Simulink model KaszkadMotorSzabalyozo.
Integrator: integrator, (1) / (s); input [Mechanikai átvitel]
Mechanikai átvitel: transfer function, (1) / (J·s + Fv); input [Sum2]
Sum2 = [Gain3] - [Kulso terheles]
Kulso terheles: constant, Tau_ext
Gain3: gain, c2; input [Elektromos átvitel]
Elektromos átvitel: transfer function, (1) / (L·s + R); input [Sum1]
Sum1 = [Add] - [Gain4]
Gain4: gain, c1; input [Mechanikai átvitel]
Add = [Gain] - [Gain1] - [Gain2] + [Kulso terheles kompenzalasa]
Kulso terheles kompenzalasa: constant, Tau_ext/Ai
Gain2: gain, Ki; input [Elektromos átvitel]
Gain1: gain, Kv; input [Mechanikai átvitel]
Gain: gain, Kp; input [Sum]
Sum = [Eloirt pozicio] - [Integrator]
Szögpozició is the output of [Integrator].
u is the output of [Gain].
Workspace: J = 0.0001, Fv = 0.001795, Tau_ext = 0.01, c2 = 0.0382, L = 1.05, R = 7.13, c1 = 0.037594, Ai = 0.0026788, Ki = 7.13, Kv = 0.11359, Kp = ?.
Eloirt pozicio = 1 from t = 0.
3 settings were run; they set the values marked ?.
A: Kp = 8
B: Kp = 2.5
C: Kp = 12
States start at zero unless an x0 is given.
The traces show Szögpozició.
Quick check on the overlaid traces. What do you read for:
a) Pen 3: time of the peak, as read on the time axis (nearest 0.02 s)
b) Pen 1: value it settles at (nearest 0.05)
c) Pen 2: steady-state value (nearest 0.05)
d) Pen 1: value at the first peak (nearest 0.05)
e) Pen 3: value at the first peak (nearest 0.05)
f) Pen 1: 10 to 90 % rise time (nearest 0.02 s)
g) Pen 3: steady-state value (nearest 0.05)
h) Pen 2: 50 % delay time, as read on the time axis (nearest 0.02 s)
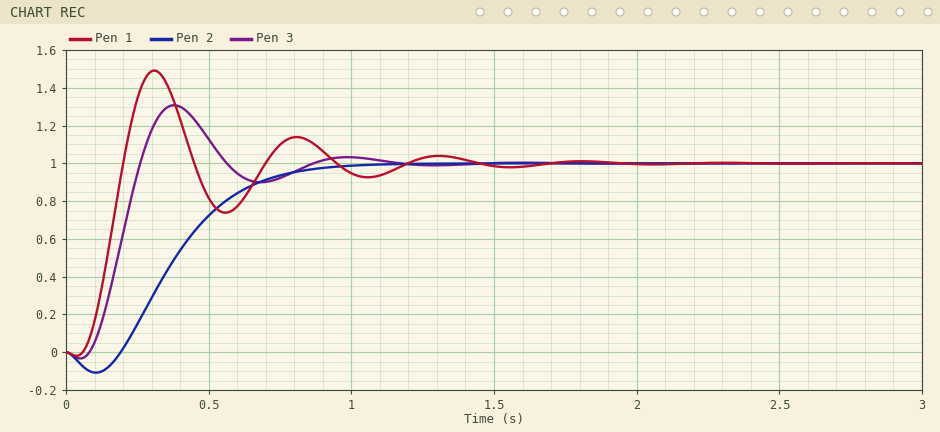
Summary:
0.38 s
1.00
1.00
1.50
1.30
0.10 s
1.00
0.38 s
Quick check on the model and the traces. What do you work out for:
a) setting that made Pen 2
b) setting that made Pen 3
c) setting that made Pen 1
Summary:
B
A
C
